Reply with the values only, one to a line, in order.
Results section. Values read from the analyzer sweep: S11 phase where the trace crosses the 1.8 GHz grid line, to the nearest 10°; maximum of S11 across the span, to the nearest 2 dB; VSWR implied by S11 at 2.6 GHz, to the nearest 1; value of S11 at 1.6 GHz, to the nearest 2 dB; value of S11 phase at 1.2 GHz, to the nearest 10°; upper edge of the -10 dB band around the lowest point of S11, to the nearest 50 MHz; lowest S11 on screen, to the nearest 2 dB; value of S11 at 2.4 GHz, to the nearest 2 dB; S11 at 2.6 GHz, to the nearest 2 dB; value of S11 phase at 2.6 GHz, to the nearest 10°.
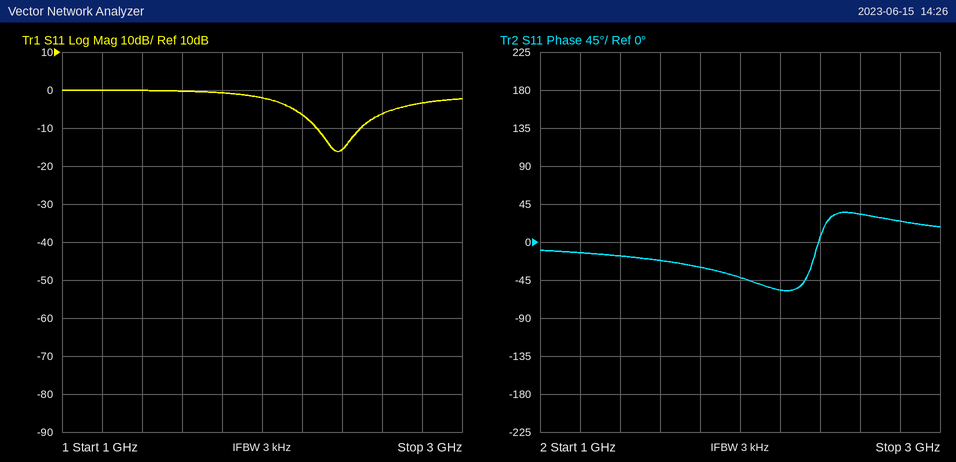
-30°
0 dB
3
0 dB
-10°
2.50 GHz
-16 dB
-16 dB
-6 dB
30°
